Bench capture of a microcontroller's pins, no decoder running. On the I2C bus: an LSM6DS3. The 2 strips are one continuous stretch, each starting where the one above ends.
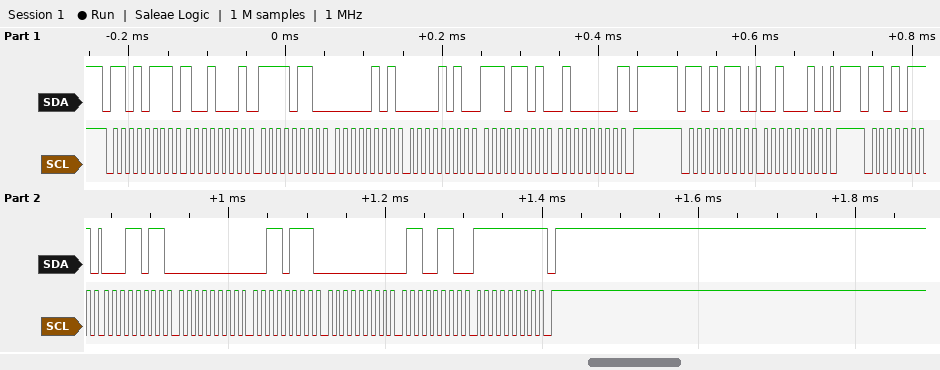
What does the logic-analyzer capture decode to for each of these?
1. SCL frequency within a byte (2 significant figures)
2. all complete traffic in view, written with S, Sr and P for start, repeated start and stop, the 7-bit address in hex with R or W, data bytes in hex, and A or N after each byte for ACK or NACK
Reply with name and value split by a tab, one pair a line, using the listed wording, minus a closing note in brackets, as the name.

SCL frequency within a byte	100 kHz
all complete traffic in view, written with S, Sr and P for start, repeated start and stop, the 7-bit address in hex with R or W, data bytes in hex, and A or N after each byte for ACK or NACK	S 6BR A 91 A F6 A 05 A 0A A ED A 40 N P S 6BW A 22 A P S 6BR A 1B A 00 A 37 A 00 A 66 A FF N P
